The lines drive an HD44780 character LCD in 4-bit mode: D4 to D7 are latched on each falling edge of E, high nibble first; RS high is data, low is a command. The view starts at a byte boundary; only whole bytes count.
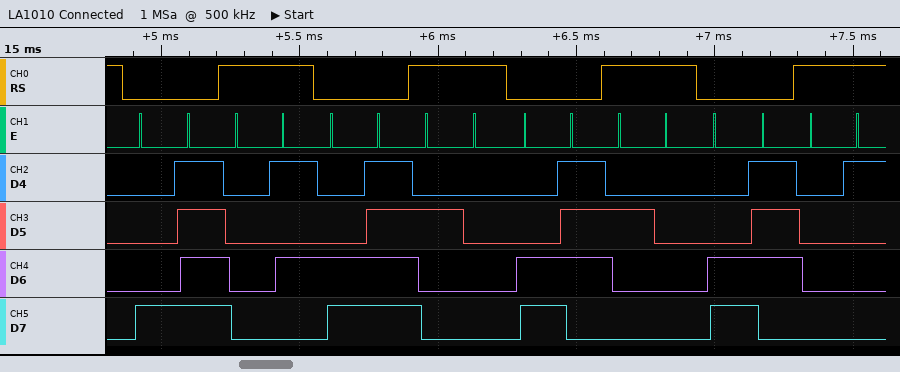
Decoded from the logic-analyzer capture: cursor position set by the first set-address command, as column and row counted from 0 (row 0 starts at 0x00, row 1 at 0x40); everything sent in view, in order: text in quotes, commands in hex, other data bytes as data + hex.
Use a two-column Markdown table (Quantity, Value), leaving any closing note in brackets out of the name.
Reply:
| Quantity | Value |
|---|---|
| cursor position set by the first set-address command, as column and row counted from 0 | column 15, row 0 |
| everything sent in view, in order: text in quotes, commands in hex, other data bytes as data + hex | 0x8F data 05 0xCF " " 0xC7 " " 0xC7 data 01 |
